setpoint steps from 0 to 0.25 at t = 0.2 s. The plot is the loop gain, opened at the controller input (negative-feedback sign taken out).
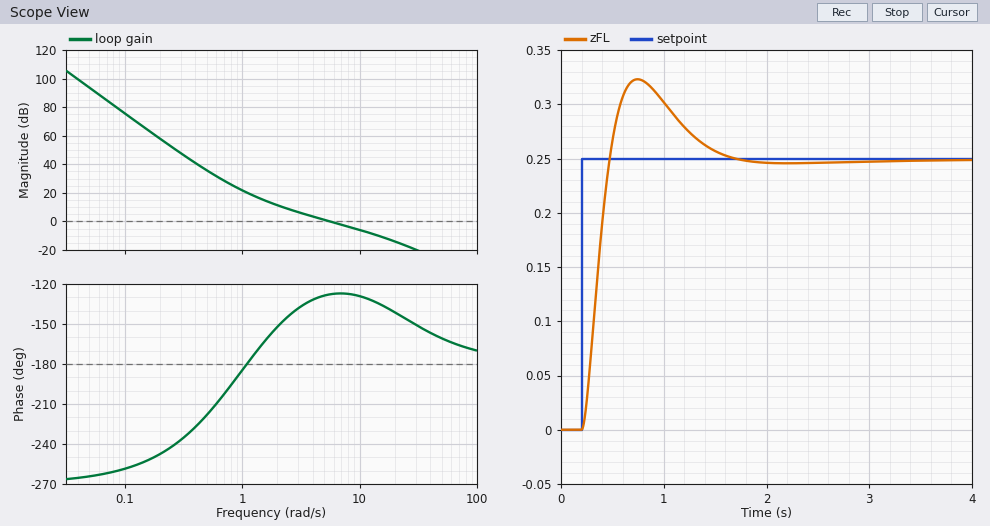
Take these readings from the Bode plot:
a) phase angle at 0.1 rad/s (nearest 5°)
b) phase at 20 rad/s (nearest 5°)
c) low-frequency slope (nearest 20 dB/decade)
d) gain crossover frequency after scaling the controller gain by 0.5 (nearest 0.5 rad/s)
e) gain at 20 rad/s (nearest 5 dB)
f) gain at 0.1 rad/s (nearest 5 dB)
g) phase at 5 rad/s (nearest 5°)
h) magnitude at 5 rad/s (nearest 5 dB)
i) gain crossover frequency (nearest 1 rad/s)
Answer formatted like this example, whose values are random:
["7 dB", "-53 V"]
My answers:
["-260°", "-140°", "-60 dB/decade", "3.0 rad/s", "-15 dB", "75 dB", "-130°", "0 dB", "6 rad/s"]
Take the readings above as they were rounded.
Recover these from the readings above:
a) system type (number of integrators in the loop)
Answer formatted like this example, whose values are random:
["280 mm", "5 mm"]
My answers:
["3"]
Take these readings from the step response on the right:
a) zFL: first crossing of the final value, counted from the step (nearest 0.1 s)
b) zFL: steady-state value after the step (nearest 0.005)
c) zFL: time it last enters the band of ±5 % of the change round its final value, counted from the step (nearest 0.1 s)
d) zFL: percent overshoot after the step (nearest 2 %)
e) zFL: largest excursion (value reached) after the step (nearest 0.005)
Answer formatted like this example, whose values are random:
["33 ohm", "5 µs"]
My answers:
["0.3 s", "0.250", "1.2 s", "30 %", "0.325"]
